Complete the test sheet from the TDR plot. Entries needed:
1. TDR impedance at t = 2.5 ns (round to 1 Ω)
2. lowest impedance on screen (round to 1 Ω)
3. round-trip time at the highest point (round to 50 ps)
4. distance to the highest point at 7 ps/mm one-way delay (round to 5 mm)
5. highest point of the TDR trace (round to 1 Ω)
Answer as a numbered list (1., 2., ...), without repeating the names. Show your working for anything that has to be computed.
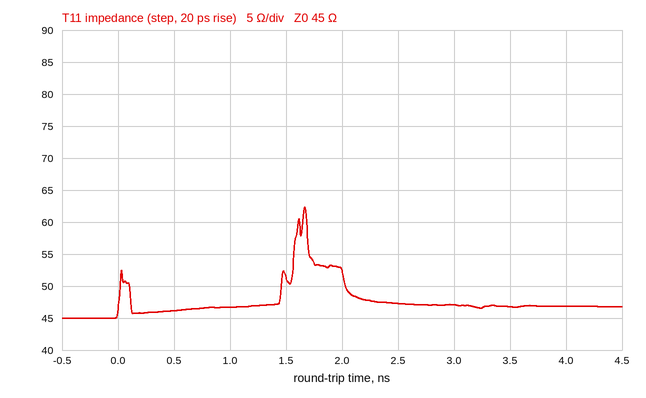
1. 47 Ω
2. 45 Ω
3. 1.65 ns
4. 1.65 ns / 2 / 7 ps/mm ≈ 118 mm, so 120 mm to the nearest 5 mm
5. 62 Ω
